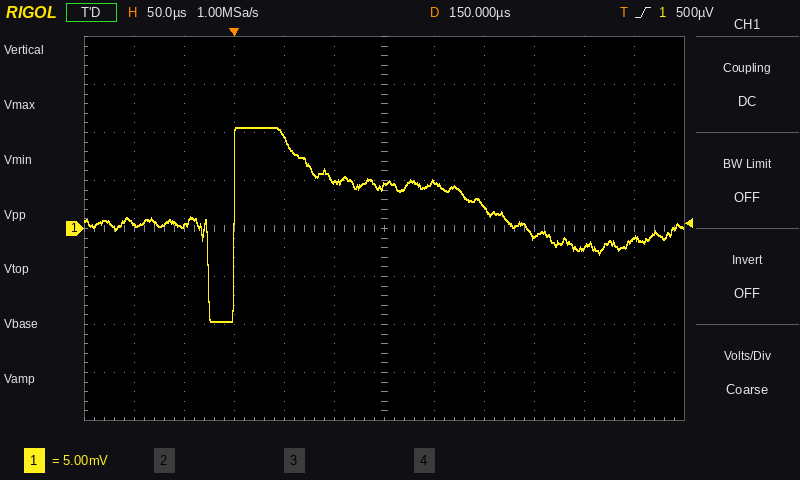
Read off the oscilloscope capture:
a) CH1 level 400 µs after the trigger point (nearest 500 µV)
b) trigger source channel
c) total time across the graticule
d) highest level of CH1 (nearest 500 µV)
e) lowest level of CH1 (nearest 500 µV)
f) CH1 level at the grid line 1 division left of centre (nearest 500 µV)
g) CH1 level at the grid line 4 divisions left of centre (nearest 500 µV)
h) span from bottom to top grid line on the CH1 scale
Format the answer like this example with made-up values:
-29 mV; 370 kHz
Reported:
-1.0 mV; CH1; 600 µs; 10.5 mV; -9.5 mV; 5.0 mV; 500 µV; 40 mV
